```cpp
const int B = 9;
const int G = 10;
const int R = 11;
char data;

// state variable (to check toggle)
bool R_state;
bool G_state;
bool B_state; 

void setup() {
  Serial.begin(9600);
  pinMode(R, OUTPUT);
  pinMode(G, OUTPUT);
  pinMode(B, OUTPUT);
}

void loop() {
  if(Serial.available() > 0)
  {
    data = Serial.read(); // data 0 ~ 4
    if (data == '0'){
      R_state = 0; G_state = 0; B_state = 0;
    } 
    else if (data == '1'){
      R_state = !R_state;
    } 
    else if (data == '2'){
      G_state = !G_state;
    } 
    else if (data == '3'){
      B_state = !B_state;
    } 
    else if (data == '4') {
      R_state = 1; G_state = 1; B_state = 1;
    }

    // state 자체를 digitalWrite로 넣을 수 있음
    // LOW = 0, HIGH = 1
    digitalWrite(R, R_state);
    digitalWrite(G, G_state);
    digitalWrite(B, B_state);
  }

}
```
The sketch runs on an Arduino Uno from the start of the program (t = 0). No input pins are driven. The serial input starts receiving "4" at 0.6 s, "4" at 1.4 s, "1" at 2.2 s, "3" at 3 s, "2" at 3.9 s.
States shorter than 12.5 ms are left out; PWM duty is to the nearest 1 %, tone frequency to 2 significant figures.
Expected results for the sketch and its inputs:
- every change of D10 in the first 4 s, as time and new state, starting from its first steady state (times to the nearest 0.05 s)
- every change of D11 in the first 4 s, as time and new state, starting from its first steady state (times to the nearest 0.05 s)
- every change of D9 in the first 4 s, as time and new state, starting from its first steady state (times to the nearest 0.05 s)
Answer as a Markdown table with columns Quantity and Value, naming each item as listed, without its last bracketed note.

| Quantity | Value |
|---|---|
| every change of D10 in the first 4 s, as time and new state, starting from its first steady state | 0 s low; 0.6 s high; 3.9 s low |
| every change of D11 in the first 4 s, as time and new state, starting from its first steady state | 0 s low; 0.6 s high; 2.2 s low |
| every change of D9 in the first 4 s, as time and new state, starting from its first steady state | 0 s low; 0.6 s high; 3 s low |
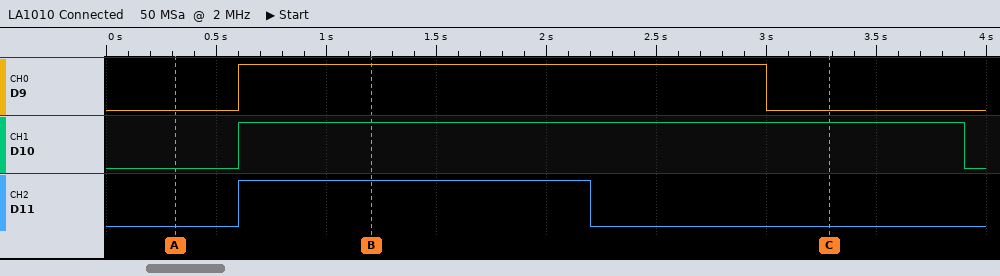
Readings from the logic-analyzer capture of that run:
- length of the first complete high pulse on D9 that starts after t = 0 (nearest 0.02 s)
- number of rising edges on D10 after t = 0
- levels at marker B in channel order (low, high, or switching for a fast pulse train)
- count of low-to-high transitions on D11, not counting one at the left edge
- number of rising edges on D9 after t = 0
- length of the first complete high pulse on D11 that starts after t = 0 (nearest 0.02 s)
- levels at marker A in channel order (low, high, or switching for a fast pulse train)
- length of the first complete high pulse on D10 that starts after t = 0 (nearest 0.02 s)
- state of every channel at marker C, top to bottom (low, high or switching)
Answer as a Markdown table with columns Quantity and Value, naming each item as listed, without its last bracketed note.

| Quantity | Value |
|---|---|
| length of the first complete high pulse on D9 that starts after t = 0 | 2.40 s |
| number of rising edges on D10 after t = 0 | 1 |
| levels at marker B in channel order | D9 high, D10 high, D11 high |
| count of low-to-high transitions on D11, not counting one at the left edge | 1 |
| number of rising edges on D9 after t = 0 | 1 |
| length of the first complete high pulse on D11 that starts after t = 0 | 1.60 s |
| levels at marker A in channel order | D9 low, D10 low, D11 low |
| length of the first complete high pulse on D10 that starts after t = 0 | 3.30 s |
| state of every channel at marker C, top to bottom | D9 low, D10 high, D11 low |
